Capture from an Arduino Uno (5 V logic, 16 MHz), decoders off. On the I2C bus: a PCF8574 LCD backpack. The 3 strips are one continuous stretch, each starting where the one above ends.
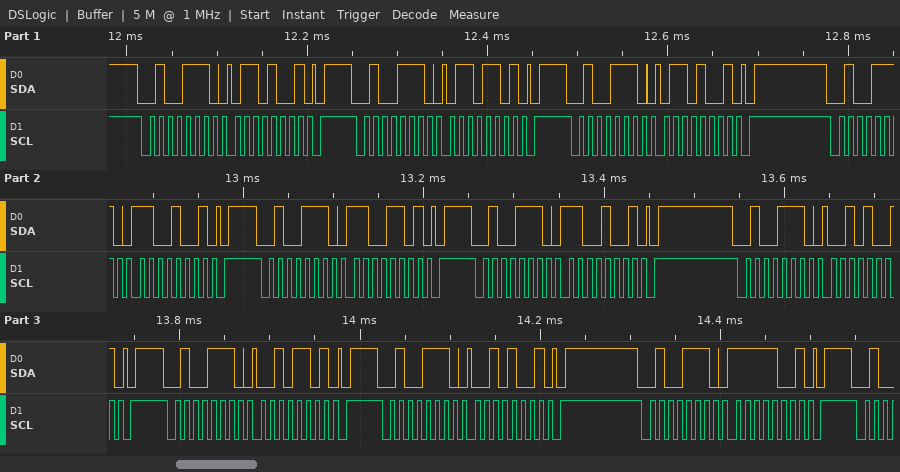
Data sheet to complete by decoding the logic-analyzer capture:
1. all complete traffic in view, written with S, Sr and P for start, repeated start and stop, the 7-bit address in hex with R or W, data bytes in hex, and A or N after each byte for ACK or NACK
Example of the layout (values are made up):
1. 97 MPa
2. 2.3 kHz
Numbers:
1. S 27W A 69 A P S 27W A 6D A P S 27W A 69 A P S 27W A C9 A P S 27W A CD A P S 27W A C9 A P S 27W A 29 A P S 27W A 2D A P S 27W A 29 A P S 27W A F9 A P
